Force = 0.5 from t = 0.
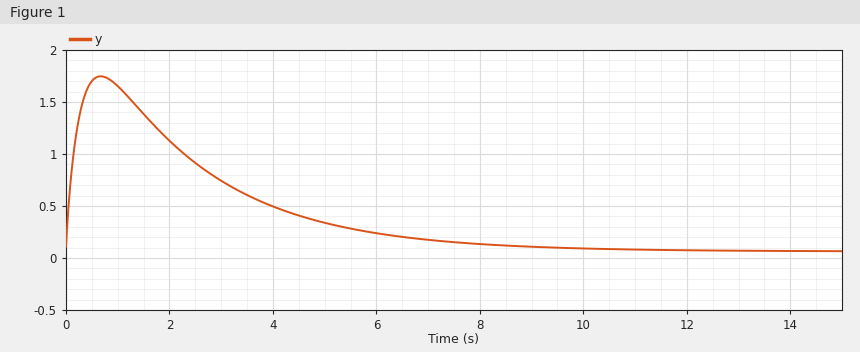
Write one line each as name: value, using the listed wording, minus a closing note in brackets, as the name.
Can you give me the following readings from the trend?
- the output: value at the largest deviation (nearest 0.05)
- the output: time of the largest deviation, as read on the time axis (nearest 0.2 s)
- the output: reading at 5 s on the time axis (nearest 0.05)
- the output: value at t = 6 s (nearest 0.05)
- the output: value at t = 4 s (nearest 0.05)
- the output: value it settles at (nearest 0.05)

the output: value at the largest deviation: 1.75
the output: time of the largest deviation, as read on the time axis: 0.6 s
the output: reading at 5 s on the time axis: 0.35
the output: value at t = 6 s: 0.25
the output: value at t = 4 s: 0.50
the output: value it settles at: 0.05
